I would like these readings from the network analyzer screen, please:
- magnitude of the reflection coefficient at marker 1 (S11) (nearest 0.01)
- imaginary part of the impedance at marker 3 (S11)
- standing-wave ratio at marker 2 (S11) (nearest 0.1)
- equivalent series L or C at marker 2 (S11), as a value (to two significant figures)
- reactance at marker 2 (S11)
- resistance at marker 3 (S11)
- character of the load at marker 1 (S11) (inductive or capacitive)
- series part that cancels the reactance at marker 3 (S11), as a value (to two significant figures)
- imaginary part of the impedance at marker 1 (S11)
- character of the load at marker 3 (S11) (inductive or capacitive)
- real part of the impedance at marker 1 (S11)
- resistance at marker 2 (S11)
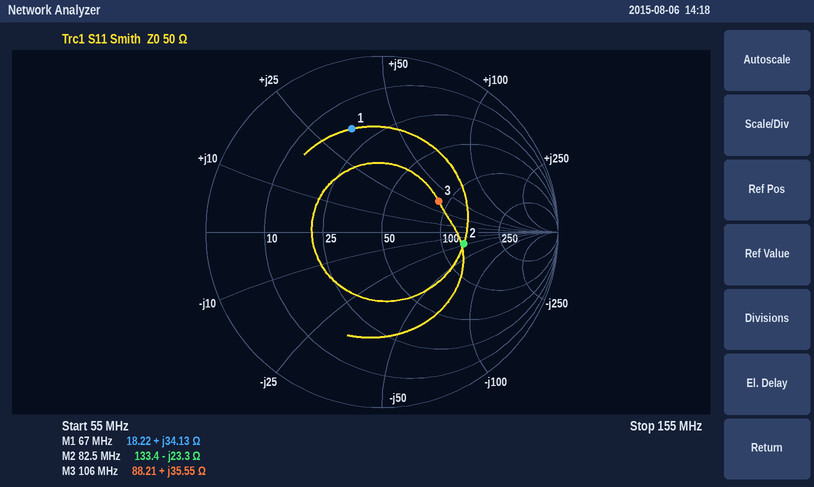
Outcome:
0.61
+35.55 Ω
2.8
83 pF
-23.3 Ω
88.21 Ω
inductive
42 pF
+34.13 Ω
inductive
18.22 Ω
133.4 Ω
